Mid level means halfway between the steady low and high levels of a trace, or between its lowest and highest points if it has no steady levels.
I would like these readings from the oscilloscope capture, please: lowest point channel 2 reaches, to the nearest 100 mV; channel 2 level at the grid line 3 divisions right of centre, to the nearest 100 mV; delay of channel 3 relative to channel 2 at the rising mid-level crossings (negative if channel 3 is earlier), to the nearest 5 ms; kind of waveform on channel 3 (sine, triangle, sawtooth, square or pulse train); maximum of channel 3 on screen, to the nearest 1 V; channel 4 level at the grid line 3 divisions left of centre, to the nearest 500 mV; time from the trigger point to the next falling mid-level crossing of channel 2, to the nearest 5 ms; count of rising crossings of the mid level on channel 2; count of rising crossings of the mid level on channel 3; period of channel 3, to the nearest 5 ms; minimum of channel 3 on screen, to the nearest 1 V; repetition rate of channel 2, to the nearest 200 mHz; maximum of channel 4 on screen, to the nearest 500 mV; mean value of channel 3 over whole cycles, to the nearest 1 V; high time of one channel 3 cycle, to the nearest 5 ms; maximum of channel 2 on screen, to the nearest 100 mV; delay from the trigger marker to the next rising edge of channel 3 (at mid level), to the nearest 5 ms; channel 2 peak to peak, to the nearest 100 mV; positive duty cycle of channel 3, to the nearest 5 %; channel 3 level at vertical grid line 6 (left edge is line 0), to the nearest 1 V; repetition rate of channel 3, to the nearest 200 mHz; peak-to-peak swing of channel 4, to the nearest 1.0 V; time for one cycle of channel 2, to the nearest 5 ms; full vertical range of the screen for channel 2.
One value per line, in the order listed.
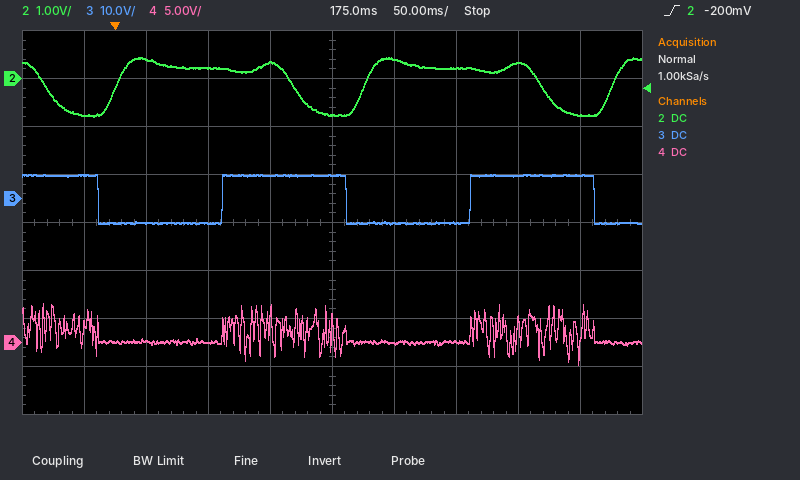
-800 mV
300 mV
+85 ms
square
5 V
0.0 V
145 ms
3
2
200 ms
-5 V
5.0 Hz
4.0 V
0 V
100 ms
400 mV
85 ms
1.2 V
50 %
-5 V
5.0 Hz
6.0 V
200 ms
8 V
